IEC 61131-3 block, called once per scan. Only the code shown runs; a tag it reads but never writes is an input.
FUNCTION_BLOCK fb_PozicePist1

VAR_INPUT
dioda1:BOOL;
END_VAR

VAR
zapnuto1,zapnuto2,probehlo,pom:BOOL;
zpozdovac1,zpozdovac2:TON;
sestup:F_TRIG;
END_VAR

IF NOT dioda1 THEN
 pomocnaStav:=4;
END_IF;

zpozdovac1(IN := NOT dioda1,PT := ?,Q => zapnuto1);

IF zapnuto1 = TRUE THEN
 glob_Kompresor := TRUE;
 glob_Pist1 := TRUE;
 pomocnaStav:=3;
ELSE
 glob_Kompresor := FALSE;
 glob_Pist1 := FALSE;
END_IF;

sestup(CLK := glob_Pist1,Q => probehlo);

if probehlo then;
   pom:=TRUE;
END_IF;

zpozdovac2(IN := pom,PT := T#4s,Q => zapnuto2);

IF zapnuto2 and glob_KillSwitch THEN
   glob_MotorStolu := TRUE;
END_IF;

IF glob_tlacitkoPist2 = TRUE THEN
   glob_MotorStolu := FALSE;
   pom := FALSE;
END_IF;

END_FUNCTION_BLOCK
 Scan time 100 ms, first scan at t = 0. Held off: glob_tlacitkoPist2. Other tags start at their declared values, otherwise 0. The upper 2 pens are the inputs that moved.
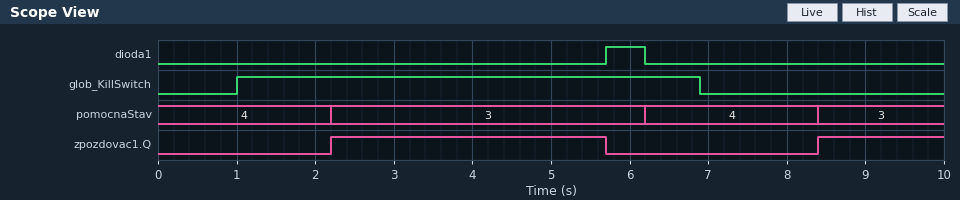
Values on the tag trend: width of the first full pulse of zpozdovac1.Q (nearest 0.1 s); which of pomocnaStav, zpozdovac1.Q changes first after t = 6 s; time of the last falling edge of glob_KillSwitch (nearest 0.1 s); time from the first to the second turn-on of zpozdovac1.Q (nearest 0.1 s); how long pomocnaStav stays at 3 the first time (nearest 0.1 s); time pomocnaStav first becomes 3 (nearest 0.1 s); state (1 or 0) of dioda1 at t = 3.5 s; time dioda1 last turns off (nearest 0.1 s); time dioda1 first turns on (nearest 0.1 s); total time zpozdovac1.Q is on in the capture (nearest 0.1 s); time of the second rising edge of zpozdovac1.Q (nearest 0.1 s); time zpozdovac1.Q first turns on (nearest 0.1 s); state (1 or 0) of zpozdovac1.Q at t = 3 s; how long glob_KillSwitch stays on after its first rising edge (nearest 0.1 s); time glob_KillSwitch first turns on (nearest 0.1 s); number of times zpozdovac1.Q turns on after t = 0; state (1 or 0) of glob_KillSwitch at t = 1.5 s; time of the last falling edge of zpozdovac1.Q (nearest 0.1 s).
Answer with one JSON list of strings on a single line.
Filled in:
["3.5 s", "pomocnaStav", "6.9 s", "6.2 s", "4.0 s", "2.2 s", "0", "6.2 s", "5.7 s", "5.1 s", "8.4 s", "2.2 s", "1", "5.9 s", "1.0 s", "2", "1", "5.7 s"]
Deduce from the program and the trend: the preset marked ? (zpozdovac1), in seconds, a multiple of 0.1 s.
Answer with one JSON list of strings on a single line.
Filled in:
["2.2 s"]
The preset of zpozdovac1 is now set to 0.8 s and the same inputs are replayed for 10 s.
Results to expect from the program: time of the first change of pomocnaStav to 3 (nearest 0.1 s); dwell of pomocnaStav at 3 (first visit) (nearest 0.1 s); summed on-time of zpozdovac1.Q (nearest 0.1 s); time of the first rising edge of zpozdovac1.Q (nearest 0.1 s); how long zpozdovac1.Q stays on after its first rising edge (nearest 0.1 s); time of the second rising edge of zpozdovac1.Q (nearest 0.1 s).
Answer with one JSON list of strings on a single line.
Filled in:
["0.8 s", "5.4 s", "7.9 s", "0.8 s", "4.9 s", "7.0 s"]
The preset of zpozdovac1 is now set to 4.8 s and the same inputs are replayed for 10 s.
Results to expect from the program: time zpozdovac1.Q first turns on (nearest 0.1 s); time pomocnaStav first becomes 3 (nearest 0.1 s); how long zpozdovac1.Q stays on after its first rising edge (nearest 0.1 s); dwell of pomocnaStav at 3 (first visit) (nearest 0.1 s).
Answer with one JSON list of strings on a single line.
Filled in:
["4.8 s", "4.8 s", "0.9 s", "1.4 s"]
